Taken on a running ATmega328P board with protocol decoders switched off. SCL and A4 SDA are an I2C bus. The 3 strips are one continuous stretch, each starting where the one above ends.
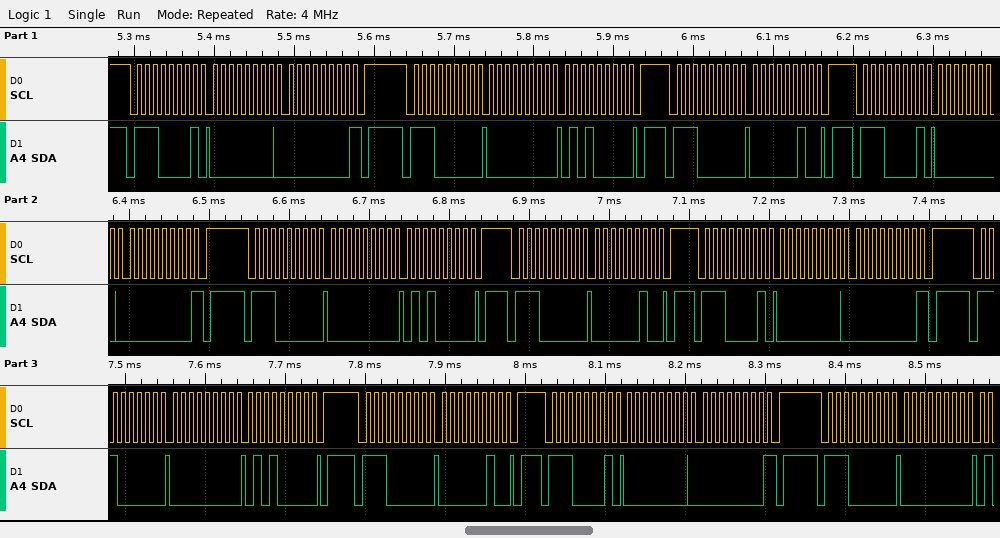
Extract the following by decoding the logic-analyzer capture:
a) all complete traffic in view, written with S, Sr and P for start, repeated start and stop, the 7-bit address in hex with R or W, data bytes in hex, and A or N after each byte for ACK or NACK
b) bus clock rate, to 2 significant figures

S 70R A 00 A 00 N P S 70W A 00 A 50 A P S 70W A 02 A P S 70R A 00 A 00 N P S 70W A 00 A 50 A P S 70W A 02 A P S 70R A 00 A 00 N P S 70W A 00 A 50 A P S 70W A 02 A P S 70R A 00 A 00 N P S 70W A 00 A
100 kHz
